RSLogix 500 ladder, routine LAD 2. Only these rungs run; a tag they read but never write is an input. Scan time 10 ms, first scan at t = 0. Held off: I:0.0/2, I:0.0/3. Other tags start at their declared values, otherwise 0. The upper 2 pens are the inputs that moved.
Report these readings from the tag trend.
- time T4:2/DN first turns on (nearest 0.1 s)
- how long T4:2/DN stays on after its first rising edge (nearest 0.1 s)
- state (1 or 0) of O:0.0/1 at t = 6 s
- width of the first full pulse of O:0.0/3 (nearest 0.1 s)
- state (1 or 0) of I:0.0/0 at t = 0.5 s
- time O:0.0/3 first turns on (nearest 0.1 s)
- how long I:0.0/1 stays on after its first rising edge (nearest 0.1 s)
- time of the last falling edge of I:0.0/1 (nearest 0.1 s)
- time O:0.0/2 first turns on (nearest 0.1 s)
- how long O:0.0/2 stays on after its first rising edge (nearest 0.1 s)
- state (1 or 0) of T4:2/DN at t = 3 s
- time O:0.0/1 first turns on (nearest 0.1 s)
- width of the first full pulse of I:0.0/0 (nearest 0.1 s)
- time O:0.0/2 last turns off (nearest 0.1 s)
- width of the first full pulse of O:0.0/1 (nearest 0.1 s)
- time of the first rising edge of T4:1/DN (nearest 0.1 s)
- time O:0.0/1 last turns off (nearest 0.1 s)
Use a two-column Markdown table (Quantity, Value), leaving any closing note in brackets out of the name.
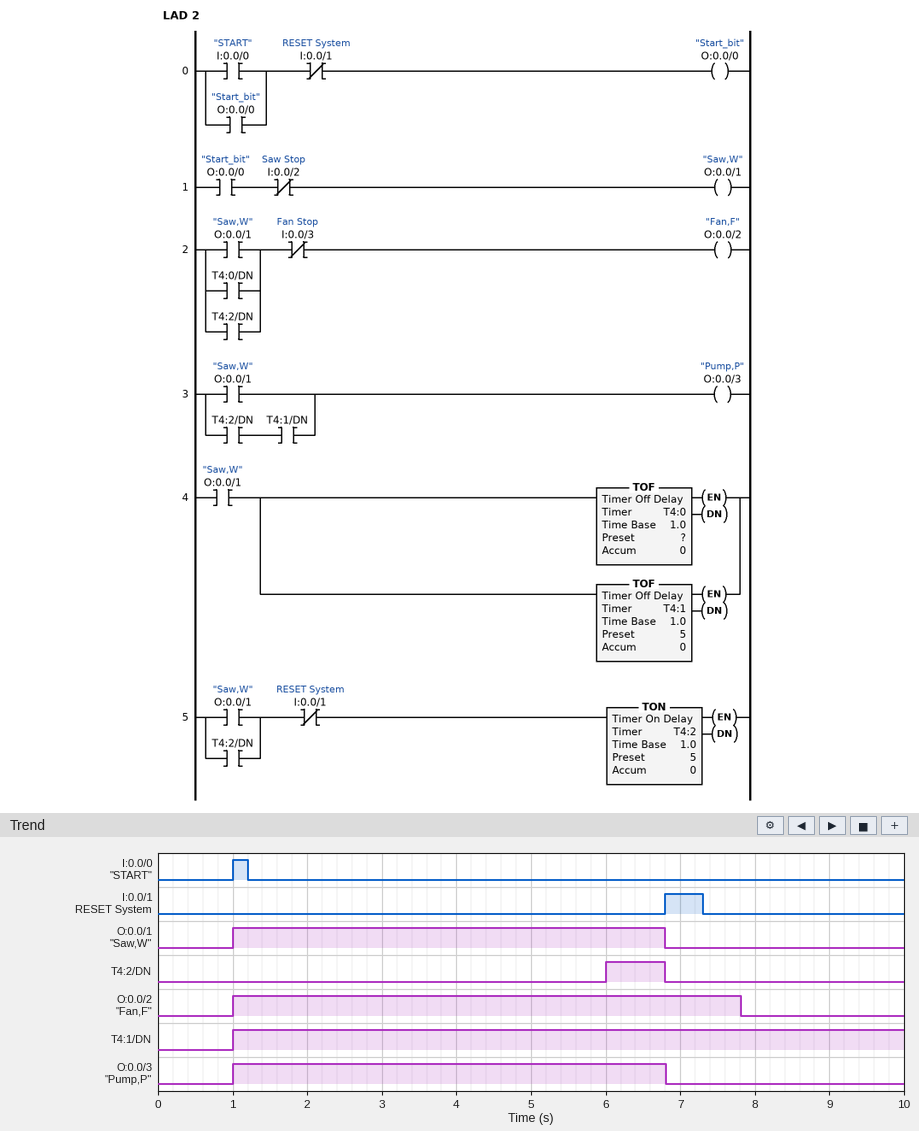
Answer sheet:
| Quantity | Value |
|---|---|
| time T4:2/DN first turns on | 6.0 s |
| how long T4:2/DN stays on after its first rising edge | 0.8 s |
| state (1 or 0) of O:0.0/1 at t = 6 s | 1 |
| width of the first full pulse of O:0.0/3 | 5.8 s |
| state (1 or 0) of I:0.0/0 at t = 0.5 s | 0 |
| time O:0.0/3 first turns on | 1.0 s |
| how long I:0.0/1 stays on after its first rising edge | 0.5 s |
| time of the last falling edge of I:0.0/1 | 7.3 s |
| time O:0.0/2 first turns on | 1.0 s |
| how long O:0.0/2 stays on after its first rising edge | 6.8 s |
| state (1 or 0) of T4:2/DN at t = 3 s | 0 |
| time O:0.0/1 first turns on | 1.0 s |
| width of the first full pulse of I:0.0/0 | 0.2 s |
| time O:0.0/2 last turns off | 7.8 s |
| width of the first full pulse of O:0.0/1 | 5.8 s |
| time of the first rising edge of T4:1/DN | 1.0 s |
| time O:0.0/1 last turns off | 6.8 s |
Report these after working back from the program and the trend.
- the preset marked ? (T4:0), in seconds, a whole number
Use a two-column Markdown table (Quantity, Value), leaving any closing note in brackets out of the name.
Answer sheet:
| Quantity | Value |
|---|---|
| the preset marked ? (T4:0), in seconds, a whole number | 1 s |
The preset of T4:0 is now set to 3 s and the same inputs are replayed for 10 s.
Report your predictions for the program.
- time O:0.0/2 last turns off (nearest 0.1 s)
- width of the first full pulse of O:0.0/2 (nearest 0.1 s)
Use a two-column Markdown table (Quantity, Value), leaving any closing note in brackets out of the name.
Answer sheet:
| Quantity | Value |
|---|---|
| time O:0.0/2 last turns off | 9.8 s |
| width of the first full pulse of O:0.0/2 | 8.8 s |
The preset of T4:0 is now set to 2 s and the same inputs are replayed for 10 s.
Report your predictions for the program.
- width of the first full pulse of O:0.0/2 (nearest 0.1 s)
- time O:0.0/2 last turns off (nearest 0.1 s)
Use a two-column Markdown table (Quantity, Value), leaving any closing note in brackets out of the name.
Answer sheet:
| Quantity | Value |
|---|---|
| width of the first full pulse of O:0.0/2 | 7.8 s |
| time O:0.0/2 last turns off | 8.8 s |
